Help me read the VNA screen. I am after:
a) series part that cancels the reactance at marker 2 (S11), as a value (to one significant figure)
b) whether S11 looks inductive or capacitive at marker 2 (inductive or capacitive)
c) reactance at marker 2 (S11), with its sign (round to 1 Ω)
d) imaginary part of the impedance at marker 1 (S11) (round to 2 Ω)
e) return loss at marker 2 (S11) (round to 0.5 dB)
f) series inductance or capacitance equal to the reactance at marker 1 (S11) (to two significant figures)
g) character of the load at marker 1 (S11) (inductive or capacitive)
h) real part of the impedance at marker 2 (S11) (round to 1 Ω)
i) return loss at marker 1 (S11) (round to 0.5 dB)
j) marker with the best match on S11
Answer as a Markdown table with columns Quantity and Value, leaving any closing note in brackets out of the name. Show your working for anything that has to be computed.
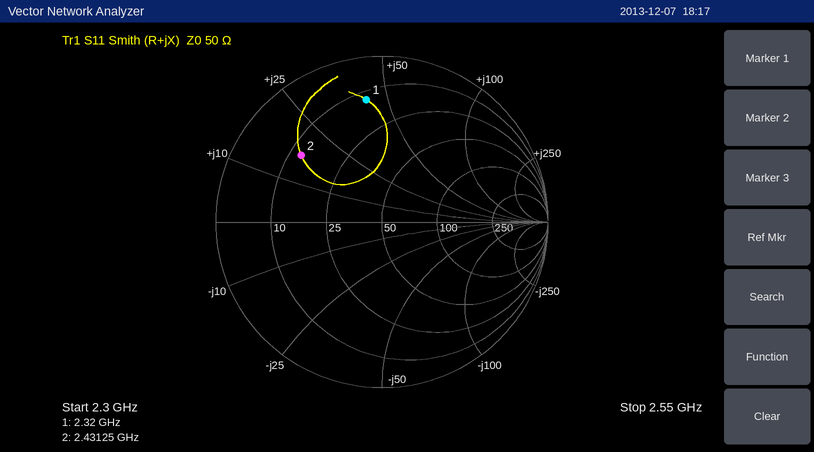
| Quantity | Value |
|---|---|
| series part that cancels the reactance at marker 2 (S11), as a value | C = 1/(2π × 2.43125 GHz × 17 Ω) ≈ 4 pF |
| whether S11 looks inductive or capacitive at marker 2 | inductive |
| reactance at marker 2 (S11), with its sign | +17 Ω |
| imaginary part of the impedance at marker 1 (S11) | +42 Ω |
| return loss at marker 2 (S11) | 4.0 dB |
| series inductance or capacitance equal to the reactance at marker 1 (S11) | L = 42 Ω/(2π × 2.32 GHz) ≈ 2.9 nH |
| character of the load at marker 1 (S11) | inductive |
| real part of the impedance at marker 2 (S11) | 13 Ω |
| return loss at marker 1 (S11) | 2.5 dB |
| marker with the best match on S11 | marker 2 |
